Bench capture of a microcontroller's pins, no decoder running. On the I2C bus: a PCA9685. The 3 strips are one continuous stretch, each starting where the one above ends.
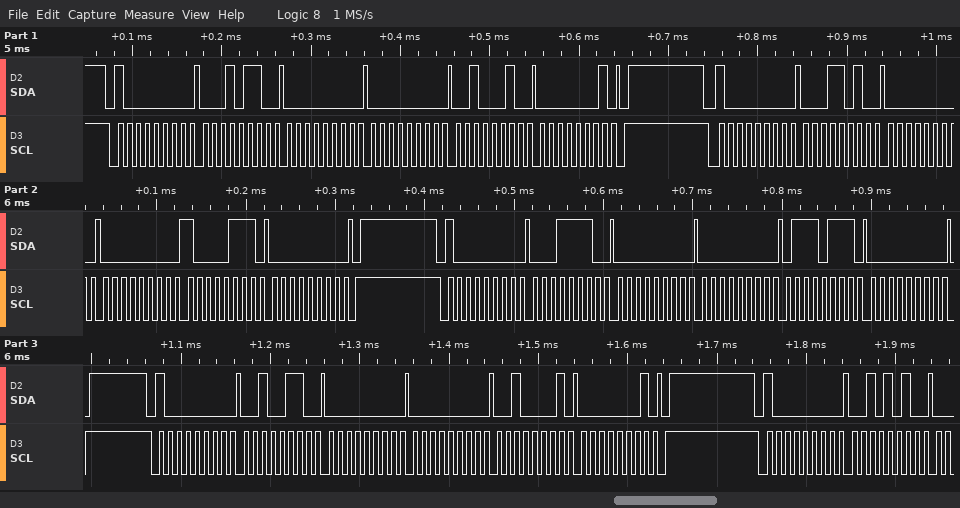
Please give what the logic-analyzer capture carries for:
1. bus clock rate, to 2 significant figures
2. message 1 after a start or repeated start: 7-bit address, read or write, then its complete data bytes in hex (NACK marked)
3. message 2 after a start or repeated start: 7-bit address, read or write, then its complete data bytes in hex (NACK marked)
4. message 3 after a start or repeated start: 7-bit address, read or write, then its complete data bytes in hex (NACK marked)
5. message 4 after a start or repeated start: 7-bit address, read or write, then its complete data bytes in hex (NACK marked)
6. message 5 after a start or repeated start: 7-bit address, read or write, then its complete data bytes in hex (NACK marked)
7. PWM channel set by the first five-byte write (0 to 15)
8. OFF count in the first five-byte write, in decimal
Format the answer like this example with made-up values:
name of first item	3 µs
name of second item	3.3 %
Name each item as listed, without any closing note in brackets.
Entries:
bus clock rate, to 2 significant figures	100 kHz
message 1 after a start or repeated start: 7-bit address, read or write, then its complete data bytes in hex	0x40 write: 16 00 00 22 01
message 2 after a start or repeated start: 7-bit address, read or write, then its complete data bytes in hex	0x40 write: 1A 00 00 87 00
message 3 after a start or repeated start: 7-bit address, read or write, then its complete data bytes in hex	0x40 write: 1E 00 00 77 00
message 4 after a start or repeated start: 7-bit address, read or write, then its complete data bytes in hex	0x40 write: 26 00 00 21 01
message 5 after a start or repeated start: 7-bit address, read or write, then its complete data bytes in hex	0x40 write: 2A
PWM channel set by the first five-byte write	4
OFF count in the first five-byte write, in decimal	290
